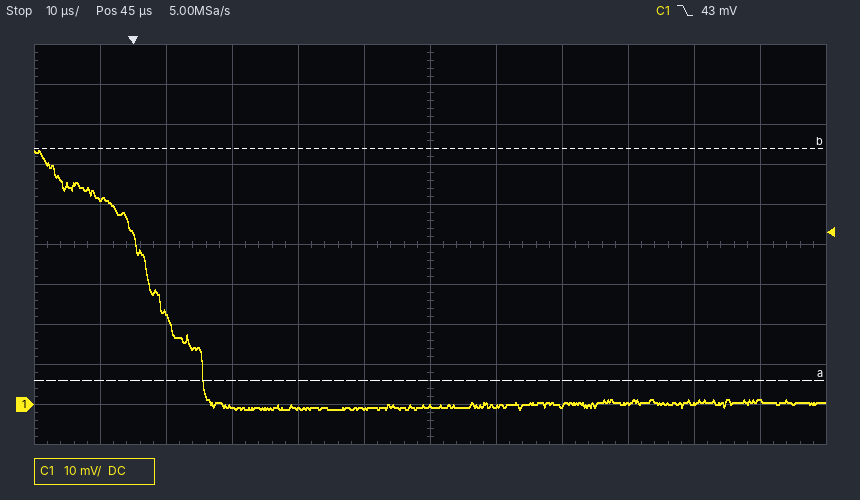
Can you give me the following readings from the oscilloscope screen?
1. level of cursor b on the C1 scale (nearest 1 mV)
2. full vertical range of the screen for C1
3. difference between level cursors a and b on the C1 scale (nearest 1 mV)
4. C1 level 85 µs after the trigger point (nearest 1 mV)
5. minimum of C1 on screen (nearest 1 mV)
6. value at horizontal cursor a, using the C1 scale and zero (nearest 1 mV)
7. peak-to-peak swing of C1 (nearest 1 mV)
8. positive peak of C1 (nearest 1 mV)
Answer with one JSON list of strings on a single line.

["64 mV", "100 mV", "58 mV", "0 mV", "-1 mV", "6 mV", "65 mV", "64 mV"]
